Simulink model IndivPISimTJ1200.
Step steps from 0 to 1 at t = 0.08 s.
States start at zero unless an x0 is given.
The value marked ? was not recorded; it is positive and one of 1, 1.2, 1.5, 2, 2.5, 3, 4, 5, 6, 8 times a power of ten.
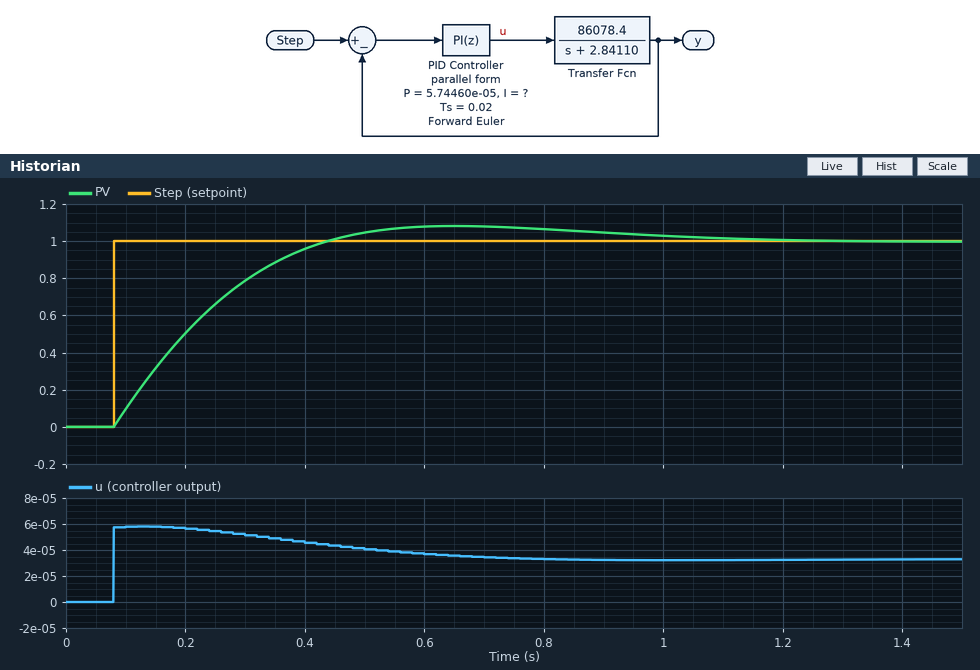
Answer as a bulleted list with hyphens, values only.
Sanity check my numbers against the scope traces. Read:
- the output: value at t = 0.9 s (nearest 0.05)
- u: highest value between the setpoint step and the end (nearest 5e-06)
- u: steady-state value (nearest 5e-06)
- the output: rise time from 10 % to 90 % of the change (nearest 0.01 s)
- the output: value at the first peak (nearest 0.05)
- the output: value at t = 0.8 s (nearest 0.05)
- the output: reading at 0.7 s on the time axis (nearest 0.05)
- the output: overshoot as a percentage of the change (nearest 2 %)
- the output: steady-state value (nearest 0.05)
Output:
- 1.05
- 0.000060
- 0.000035
- 0.26 s
- 1.10
- 1.05
- 1.10
- 8 %
- 1.00
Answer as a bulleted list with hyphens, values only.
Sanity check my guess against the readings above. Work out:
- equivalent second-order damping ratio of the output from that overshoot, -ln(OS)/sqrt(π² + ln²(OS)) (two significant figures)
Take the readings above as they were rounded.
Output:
- 0.63
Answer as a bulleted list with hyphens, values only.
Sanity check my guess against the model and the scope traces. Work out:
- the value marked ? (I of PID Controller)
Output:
- 0.0003
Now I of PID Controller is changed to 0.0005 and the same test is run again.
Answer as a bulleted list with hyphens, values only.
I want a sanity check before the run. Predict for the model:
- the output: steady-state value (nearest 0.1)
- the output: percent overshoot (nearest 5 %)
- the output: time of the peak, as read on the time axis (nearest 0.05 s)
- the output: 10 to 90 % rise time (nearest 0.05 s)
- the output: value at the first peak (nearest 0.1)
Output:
- 1.0
- 20 %
- 0.50 s
- 0.20 s
- 1.2
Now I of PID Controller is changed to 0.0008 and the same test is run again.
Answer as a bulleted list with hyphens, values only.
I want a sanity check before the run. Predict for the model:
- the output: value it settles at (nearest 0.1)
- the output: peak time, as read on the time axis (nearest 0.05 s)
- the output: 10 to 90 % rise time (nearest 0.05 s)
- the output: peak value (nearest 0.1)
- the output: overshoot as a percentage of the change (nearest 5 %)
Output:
- 1.0
- 0.40 s
- 0.15 s
- 1.3
- 30 %
